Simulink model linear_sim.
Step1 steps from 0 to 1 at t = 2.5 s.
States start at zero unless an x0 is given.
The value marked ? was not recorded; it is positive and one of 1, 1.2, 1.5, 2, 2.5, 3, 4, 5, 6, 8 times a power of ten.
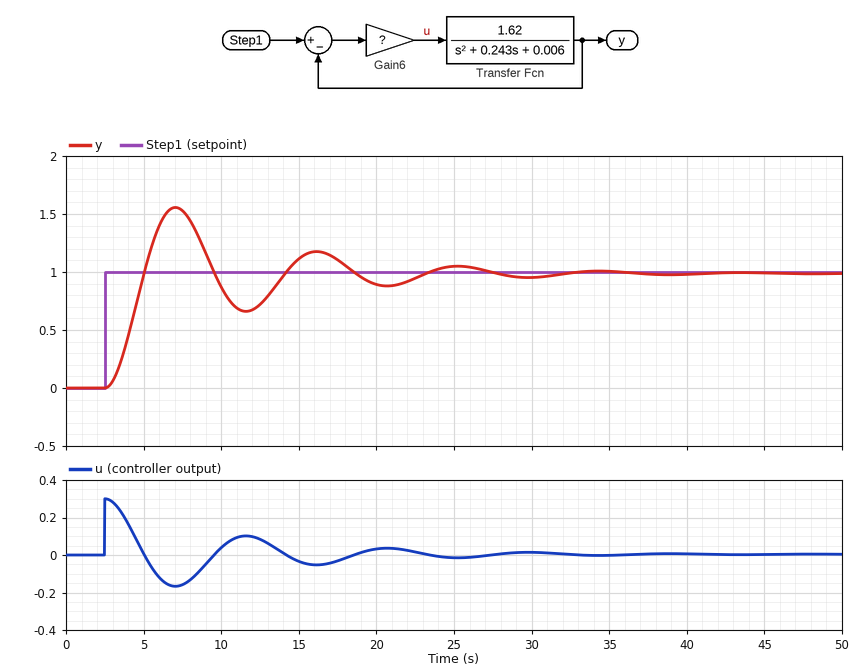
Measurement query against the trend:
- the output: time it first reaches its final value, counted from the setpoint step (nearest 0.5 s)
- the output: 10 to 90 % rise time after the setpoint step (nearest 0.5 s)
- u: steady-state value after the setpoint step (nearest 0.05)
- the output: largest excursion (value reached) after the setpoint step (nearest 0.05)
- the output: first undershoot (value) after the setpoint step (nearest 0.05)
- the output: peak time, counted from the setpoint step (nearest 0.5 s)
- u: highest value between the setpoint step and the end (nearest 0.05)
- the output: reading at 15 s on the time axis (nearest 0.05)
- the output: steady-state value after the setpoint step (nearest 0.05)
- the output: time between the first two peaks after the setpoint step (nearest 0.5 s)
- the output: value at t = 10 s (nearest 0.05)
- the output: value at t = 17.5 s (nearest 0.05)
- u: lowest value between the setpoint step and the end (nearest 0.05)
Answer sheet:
2.5 s
1.5 s
0.00
1.55
0.65
4.5 s
0.30
1.10
1.00
9.0 s
0.85
1.10
-0.15
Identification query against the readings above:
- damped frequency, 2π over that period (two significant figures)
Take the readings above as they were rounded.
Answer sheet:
0.70 rad/s
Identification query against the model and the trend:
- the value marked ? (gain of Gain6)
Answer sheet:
0.3
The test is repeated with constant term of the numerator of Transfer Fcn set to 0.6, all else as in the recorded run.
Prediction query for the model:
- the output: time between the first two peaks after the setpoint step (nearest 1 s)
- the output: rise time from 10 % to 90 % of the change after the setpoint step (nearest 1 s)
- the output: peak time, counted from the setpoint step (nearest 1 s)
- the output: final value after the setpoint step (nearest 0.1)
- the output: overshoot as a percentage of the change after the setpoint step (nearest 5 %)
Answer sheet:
15 s
3 s
8 s
1.0
40 %
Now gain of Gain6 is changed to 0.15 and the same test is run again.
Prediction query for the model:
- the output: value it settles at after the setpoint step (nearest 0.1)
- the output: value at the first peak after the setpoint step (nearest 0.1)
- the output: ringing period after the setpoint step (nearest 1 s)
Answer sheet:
1.0
1.4
13 s
